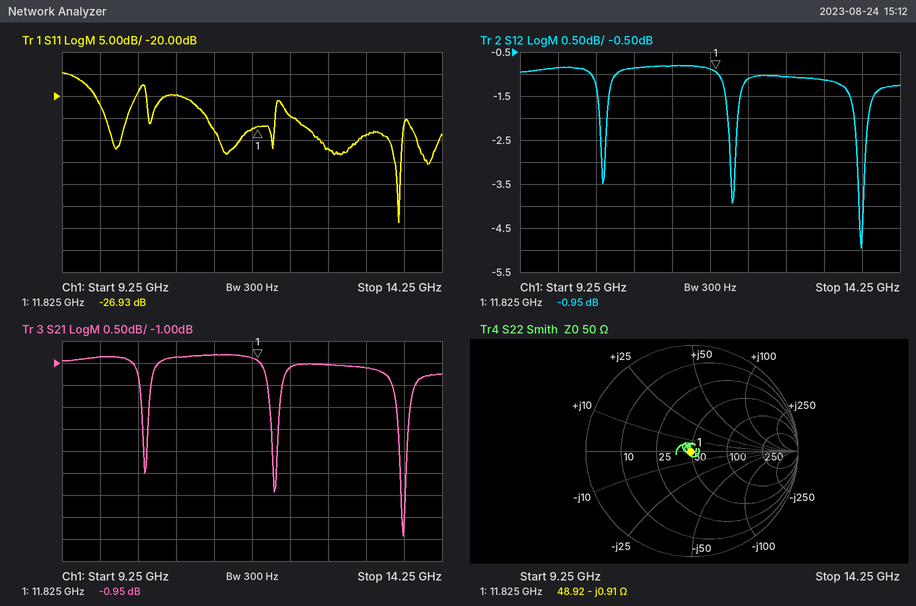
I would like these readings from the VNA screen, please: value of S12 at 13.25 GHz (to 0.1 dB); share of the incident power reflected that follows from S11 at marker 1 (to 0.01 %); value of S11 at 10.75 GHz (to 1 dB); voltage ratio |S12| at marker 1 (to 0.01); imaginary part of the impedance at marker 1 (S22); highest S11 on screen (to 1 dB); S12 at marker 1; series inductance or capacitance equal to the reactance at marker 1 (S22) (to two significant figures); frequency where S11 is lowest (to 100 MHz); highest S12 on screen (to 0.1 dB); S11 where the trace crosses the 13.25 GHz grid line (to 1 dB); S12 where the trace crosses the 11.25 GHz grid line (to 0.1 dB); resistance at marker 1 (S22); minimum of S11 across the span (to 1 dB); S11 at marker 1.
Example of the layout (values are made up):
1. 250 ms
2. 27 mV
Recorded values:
1. -1.1 dB
2. 0.20 %
3. -20 dB
4. 0.90
5. -0.91 Ω
6. -15 dB
7. -0.95 dB
8. 15 pF
9. 13.7 GHz
10. -0.8 dB
11. -29 dB
12. -0.8 dB
13. 48.92 Ω
14. -49 dB
15. -26.93 dB
